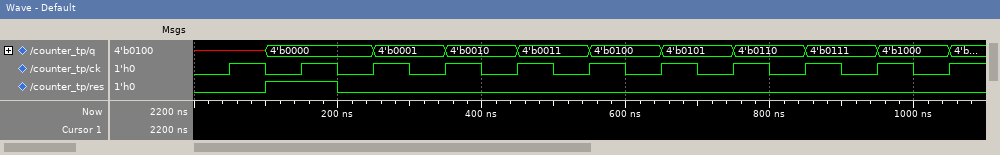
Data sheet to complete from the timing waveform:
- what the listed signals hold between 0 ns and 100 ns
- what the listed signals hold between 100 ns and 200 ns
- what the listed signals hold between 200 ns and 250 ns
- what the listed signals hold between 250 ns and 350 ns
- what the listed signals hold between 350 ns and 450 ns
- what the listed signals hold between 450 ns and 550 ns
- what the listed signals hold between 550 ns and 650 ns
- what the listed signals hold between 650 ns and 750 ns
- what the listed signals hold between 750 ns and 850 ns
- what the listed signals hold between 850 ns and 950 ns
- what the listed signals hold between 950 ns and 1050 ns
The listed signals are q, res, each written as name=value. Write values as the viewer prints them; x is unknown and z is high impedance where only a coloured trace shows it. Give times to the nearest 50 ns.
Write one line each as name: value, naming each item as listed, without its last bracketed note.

what the listed signals hold between 0 ns and 100 ns: q=x, res=0
what the listed signals hold between 100 ns and 200 ns: q=4'b0000, res=1
what the listed signals hold between 200 ns and 250 ns: q=4'b0000, res=0
what the listed signals hold between 250 ns and 350 ns: q=4'b0001, res=0
what the listed signals hold between 350 ns and 450 ns: q=4'b0010, res=0
what the listed signals hold between 450 ns and 550 ns: q=4'b0011, res=0
what the listed signals hold between 550 ns and 650 ns: q=4'b0100, res=0
what the listed signals hold between 650 ns and 750 ns: q=4'b0101, res=0
what the listed signals hold between 750 ns and 850 ns: q=4'b0110, res=0
what the listed signals hold between 850 ns and 950 ns: q=4'b0111, res=0
what the listed signals hold between 950 ns and 1050 ns: q=4'b1000, res=0
